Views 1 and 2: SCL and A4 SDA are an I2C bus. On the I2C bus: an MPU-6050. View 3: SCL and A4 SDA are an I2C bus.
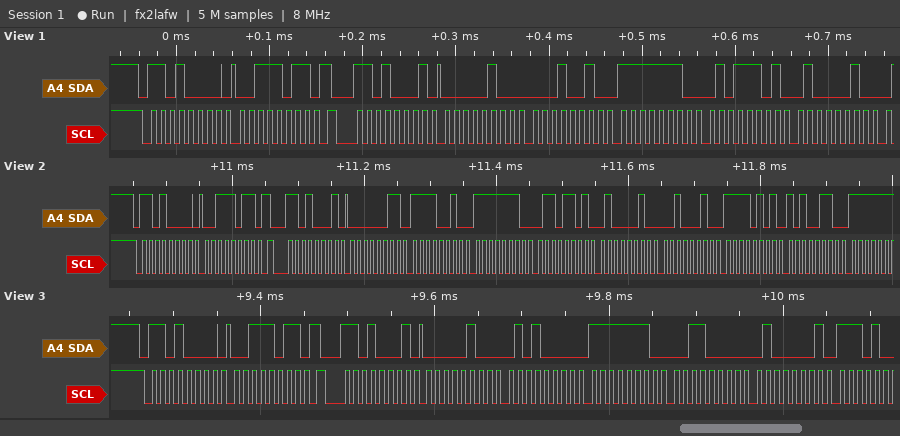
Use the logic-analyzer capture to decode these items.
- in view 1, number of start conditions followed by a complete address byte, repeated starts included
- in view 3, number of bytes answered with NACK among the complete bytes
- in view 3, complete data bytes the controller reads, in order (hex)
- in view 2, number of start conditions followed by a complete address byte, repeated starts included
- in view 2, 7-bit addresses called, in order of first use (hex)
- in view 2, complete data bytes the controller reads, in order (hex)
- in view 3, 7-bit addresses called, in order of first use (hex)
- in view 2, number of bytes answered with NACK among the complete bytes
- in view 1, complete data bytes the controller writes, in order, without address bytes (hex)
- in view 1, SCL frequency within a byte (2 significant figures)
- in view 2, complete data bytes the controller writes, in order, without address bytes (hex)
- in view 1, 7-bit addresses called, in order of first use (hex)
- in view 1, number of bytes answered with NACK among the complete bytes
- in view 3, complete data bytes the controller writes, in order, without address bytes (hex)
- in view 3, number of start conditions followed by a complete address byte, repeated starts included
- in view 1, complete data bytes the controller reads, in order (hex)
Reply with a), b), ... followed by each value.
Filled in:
a) 2
b) 0
c) 04 50 FE 30 41
d) 2
e) 0x68
f) 03 F2 FE 6D 42 22 F5 A6
g) 0x68
h) 0
i) 3B
j) 100 kHz
k) 3B
l) 0x68
m) 0
n) 3B
o) 2
p) 04 12 FE 5D 42
